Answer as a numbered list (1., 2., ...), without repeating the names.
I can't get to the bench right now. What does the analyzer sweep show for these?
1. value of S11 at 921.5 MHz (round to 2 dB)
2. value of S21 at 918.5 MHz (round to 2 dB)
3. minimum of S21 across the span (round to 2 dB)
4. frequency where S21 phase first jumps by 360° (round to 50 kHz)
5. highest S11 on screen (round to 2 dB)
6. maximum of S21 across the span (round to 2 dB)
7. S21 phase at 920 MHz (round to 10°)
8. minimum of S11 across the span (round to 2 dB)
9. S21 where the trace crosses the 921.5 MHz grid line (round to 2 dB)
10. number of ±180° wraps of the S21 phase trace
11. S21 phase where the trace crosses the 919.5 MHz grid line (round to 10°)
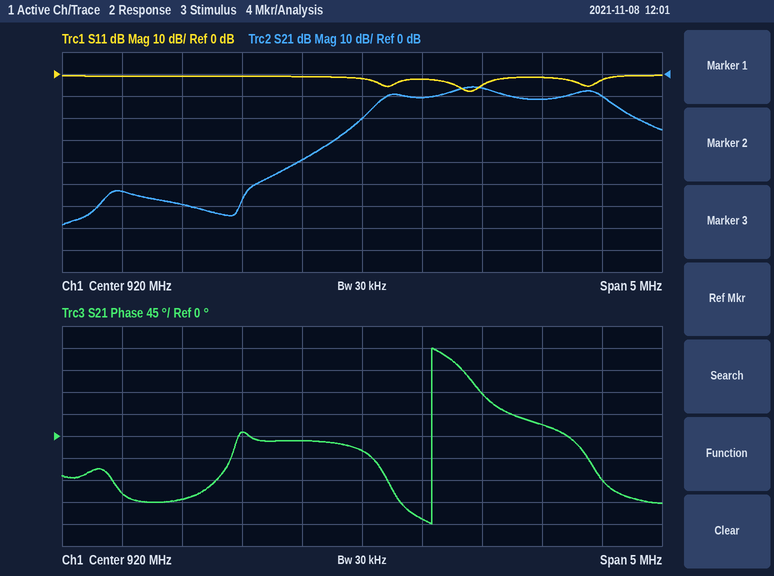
1. -2 dB
2. -60 dB
3. -68 dB
4. 920.60 MHz
5. 0 dB
6. -6 dB
7. -30°
8. -8 dB
9. -12 dB
10. 1
11. -10°
